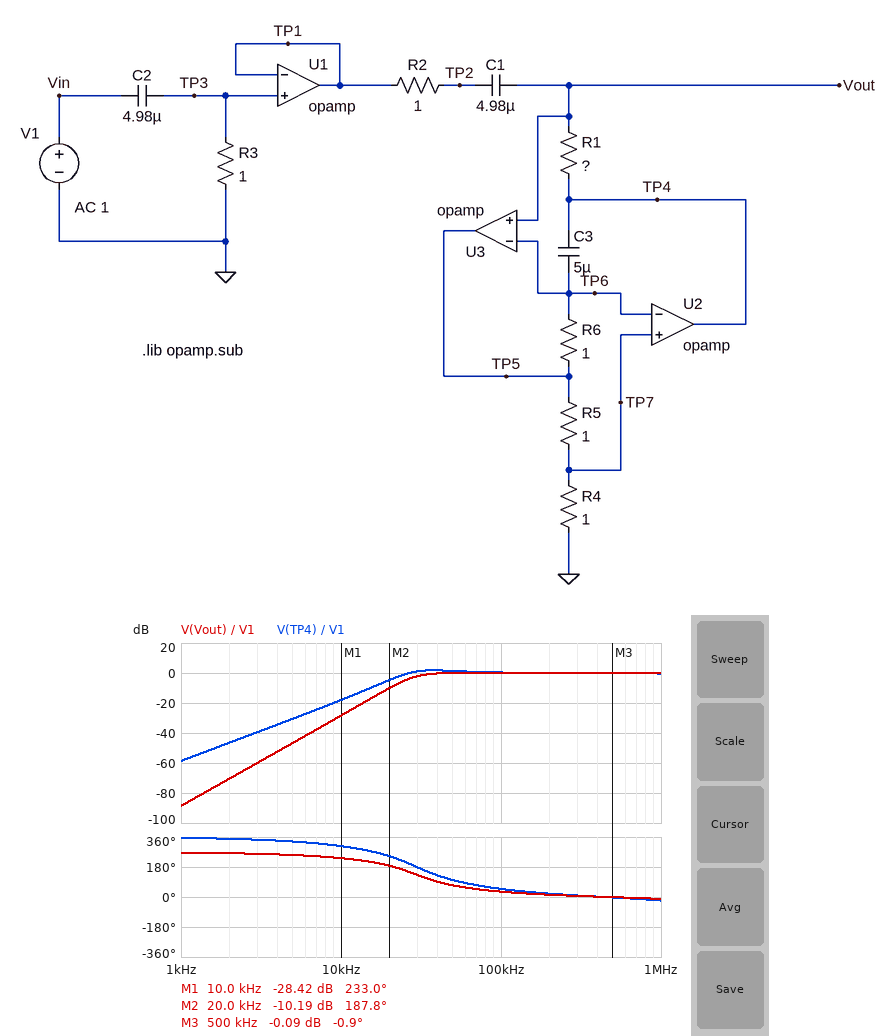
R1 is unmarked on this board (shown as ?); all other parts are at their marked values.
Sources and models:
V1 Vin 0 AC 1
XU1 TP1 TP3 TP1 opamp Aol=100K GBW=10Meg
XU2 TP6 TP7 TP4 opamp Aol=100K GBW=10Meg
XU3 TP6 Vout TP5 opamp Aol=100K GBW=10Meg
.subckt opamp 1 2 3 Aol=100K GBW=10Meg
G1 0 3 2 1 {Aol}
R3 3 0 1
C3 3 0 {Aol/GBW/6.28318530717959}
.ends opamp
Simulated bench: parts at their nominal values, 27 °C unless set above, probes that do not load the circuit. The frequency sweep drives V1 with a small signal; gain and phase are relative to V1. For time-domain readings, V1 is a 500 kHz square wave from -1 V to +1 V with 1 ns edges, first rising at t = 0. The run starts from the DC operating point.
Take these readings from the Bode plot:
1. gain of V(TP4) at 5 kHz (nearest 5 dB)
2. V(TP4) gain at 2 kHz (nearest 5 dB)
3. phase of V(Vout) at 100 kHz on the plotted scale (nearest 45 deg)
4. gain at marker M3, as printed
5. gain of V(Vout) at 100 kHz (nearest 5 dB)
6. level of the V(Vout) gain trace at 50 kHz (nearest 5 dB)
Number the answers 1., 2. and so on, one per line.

1. -30 dB
2. -45 dB
3. 45 deg
4. -0.09 dB
5. 0 dB
6. 0 dB
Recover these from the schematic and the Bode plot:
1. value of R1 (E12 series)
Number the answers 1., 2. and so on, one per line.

1. 1.2 Ω
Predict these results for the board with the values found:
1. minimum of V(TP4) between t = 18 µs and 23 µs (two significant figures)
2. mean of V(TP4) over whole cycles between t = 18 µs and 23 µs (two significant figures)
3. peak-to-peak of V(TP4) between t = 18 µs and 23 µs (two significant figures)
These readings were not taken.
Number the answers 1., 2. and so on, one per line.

1. -920 mV
2. 260 mV
3. 2.4 V
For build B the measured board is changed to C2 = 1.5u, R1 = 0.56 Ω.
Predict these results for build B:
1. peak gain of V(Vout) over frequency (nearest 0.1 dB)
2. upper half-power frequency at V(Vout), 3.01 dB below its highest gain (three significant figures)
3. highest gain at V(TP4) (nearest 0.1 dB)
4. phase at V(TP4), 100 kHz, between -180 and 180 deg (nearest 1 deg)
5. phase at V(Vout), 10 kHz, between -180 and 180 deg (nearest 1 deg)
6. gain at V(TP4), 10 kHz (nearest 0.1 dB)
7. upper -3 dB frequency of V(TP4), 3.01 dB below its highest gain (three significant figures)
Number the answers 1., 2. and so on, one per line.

1. -0.3 dB
2. 2.26 MHz
3. -0.4 dB
4. 95 deg
5. -114 deg
6. -35.2 dB
7. 2.24 MHz
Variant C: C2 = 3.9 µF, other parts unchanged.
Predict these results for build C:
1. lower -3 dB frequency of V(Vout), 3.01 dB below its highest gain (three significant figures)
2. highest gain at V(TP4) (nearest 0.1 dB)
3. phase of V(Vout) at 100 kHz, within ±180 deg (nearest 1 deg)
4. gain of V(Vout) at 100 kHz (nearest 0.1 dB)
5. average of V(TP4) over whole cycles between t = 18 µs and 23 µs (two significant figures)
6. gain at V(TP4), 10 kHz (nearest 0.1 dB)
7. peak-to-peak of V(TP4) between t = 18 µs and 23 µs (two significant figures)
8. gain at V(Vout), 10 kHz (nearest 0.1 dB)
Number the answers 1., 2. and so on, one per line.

1. 30.8 kHz
2. 0.8 dB
3. 37 deg
4. -0.3 dB
5. 240 mV
6. -20.0 dB
7. 2.4 V
8. -30.4 dB
